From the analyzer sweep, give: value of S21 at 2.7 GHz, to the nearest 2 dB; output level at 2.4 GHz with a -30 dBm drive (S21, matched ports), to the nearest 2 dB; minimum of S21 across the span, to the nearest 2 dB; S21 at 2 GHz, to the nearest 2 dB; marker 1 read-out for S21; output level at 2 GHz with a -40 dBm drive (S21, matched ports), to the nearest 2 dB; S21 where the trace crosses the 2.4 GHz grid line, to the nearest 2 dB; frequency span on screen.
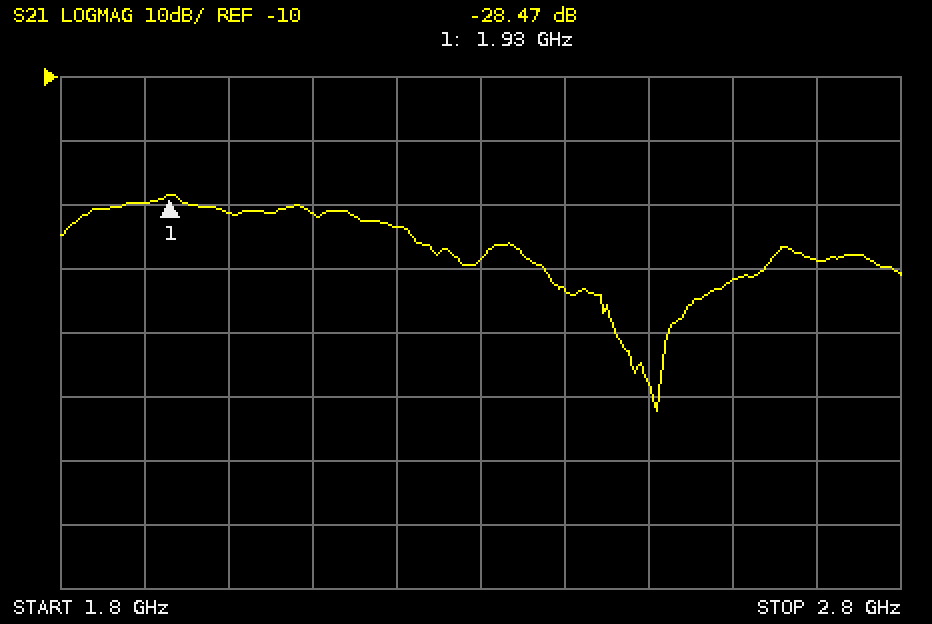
-38 dB
-74 dBm
-62 dB
-32 dB
-28.47 dB
-72 dBm
-44 dB
1 GHz
